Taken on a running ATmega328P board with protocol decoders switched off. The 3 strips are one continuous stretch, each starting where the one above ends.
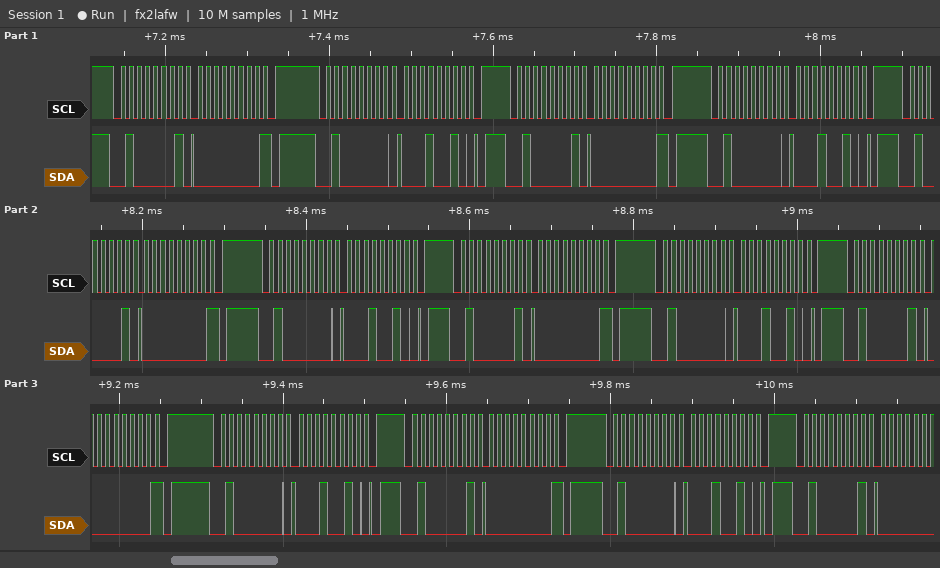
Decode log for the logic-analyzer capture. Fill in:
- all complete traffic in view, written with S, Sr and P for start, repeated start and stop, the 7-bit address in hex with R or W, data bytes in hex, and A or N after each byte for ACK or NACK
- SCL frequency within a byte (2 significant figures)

S 20R A 00 N P S 20W A 12 A P S 20R A 00 N P S 20W A 12 A P S 20R A 00 N P S 20W A 12 A P S 20R A 00 N P S 20W A 12 A P S 20R A 00 N P S 20W A 12 A P S 20R A 00 N P S 20W A 12 A P S 20R A
100 kHz
